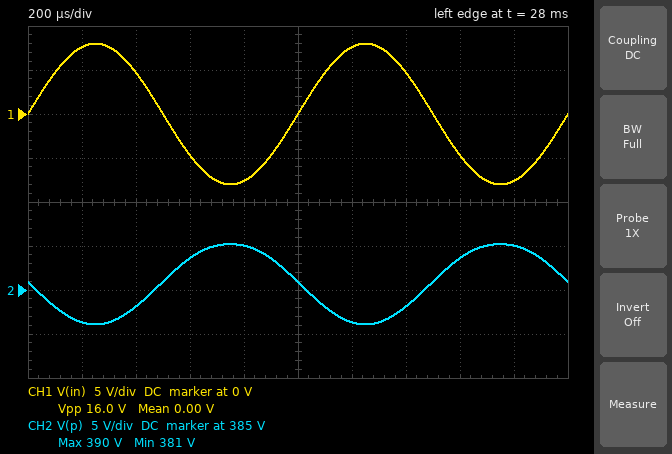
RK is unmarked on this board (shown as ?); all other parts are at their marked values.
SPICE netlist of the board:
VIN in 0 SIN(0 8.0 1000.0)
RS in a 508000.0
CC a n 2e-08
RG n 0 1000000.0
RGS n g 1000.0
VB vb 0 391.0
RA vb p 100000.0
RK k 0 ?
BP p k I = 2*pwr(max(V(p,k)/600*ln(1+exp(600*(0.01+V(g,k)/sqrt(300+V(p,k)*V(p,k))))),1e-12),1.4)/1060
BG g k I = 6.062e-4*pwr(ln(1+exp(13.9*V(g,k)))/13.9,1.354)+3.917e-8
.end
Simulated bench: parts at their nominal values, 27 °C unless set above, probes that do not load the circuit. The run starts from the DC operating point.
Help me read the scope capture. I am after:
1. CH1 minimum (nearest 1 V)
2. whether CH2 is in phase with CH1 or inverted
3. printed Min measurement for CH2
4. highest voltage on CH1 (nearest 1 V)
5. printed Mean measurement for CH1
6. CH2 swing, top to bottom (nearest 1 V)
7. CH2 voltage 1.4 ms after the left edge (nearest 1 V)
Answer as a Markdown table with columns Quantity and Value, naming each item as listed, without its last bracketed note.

| Quantity | Value |
|---|---|
| CH1 minimum | -8 V |
| whether CH2 is in phase with CH1 or inverted | inverted |
| printed Min measurement for CH2 | 381 V |
| highest voltage on CH1 | 8 V |
| printed Mean measurement for CH1 | 0.00 V |
| CH2 swing, top to bottom | 9 V |
| CH2 voltage 1.4 ms after the left edge | 383 V |
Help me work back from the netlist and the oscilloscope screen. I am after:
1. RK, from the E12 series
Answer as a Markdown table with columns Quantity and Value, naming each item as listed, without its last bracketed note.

| Quantity | Value |
|---|---|
| RK, from the E12 series | 100 kΩ |
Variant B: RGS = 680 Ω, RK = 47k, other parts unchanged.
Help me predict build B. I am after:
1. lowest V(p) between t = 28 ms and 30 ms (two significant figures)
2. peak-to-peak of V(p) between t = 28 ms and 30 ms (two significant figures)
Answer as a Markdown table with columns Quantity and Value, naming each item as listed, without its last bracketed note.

| Quantity | Value |
|---|---|
| lowest V(p) between t = 28 ms and 30 ms | 370 V |
| peak-to-peak of V(p) between t = 28 ms and 30 ms | 19 V |
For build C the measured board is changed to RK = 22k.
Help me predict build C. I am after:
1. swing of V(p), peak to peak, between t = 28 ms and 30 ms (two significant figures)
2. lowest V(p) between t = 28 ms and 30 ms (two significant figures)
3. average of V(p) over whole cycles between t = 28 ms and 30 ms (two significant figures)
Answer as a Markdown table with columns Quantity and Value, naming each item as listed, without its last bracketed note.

| Quantity | Value |
|---|---|
| swing of V(p), peak to peak, between t = 28 ms and 30 ms | 38 V |
| lowest V(p) between t = 28 ms and 30 ms | 350 V |
| average of V(p) over whole cycles between t = 28 ms and 30 ms | 370 V |
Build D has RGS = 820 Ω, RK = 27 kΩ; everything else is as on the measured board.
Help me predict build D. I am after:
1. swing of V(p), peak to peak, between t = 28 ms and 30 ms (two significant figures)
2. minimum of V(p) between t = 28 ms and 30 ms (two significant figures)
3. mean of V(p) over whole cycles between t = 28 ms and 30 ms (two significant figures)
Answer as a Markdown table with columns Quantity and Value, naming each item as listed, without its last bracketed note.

| Quantity | Value |
|---|---|
| swing of V(p), peak to peak, between t = 28 ms and 30 ms | 32 V |
| minimum of V(p) between t = 28 ms and 30 ms | 360 V |
| mean of V(p) over whole cycles between t = 28 ms and 30 ms | 370 V |
